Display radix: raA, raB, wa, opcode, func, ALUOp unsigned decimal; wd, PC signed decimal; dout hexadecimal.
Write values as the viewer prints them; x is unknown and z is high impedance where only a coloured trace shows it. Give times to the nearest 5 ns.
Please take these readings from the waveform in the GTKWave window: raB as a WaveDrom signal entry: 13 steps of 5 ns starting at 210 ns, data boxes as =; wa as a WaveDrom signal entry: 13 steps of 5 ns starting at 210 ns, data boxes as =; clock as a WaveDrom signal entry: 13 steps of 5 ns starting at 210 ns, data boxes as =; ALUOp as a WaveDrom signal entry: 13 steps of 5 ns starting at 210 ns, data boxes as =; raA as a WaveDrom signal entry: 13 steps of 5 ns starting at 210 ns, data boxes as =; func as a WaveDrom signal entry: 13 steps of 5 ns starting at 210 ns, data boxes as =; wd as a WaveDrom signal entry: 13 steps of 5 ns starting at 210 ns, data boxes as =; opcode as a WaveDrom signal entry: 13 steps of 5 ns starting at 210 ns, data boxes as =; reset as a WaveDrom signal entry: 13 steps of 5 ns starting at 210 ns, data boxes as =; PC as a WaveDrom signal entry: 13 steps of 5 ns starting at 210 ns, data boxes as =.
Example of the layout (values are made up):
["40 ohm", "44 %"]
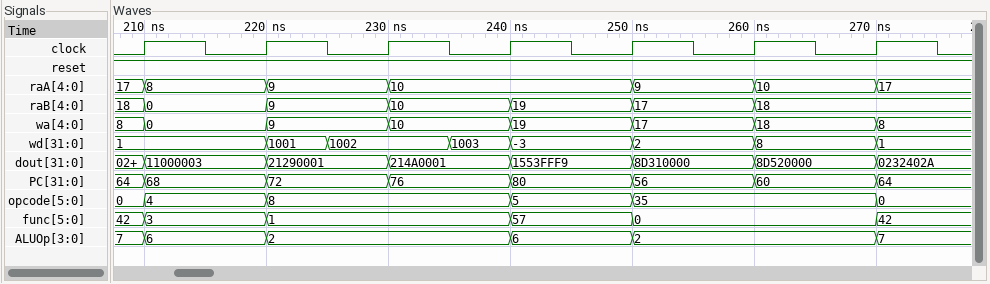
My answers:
["{name: 'raB', wave: '=.=.=.=.=.=..', data: '0 9 10 19 17 18'}", "{name: 'wa', wave: '=.=.=.=.=.=.=', data: '0 9 10 19 17 18 8'}", "{name: 'clock', wave: '1010101010101'}", "{name: 'ALUOp', wave: '=.=...=.=...=', data: '6 2 6 2 7'}", "{name: 'raA', wave: '=.=.=...=.=.=', data: '8 9 10 9 10 17'}", "{name: 'func', wave: '=.=...=.=...=', data: '3 1 57 0 42'}", "{name: 'wd', wave: '=.==.==.=.=.=', data: '1 1001 1002 1003 -3 2 8 1'}", "{name: 'opcode', wave: '=.=...=.=...=', data: '4 8 5 35 0'}", "{name: 'reset', wave: '1............'}", "{name: 'PC', wave: '=.=.=.=.=.=.=', data: '68 72 76 80 56 60 64'}"]
